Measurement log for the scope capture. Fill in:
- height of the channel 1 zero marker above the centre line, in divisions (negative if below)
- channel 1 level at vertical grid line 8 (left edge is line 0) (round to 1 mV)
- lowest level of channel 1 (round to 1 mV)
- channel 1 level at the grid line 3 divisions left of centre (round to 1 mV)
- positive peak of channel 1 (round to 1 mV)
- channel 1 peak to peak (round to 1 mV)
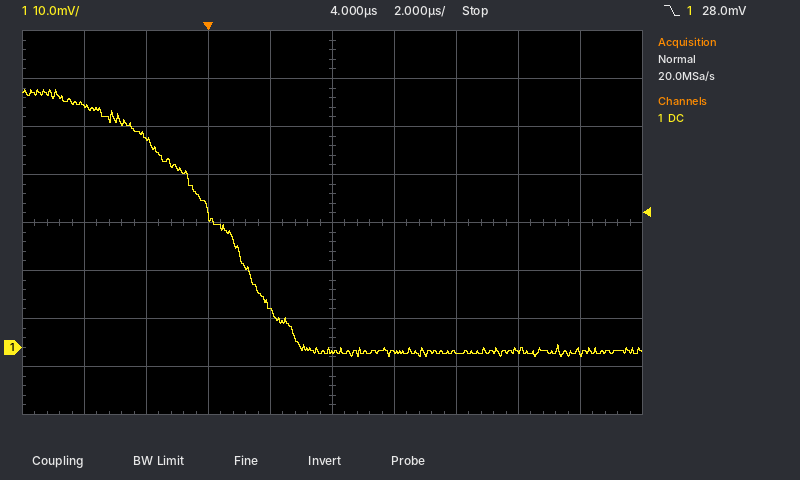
-2.6 div
-1 mV
-2 mV
44 mV
54 mV
56 mV
